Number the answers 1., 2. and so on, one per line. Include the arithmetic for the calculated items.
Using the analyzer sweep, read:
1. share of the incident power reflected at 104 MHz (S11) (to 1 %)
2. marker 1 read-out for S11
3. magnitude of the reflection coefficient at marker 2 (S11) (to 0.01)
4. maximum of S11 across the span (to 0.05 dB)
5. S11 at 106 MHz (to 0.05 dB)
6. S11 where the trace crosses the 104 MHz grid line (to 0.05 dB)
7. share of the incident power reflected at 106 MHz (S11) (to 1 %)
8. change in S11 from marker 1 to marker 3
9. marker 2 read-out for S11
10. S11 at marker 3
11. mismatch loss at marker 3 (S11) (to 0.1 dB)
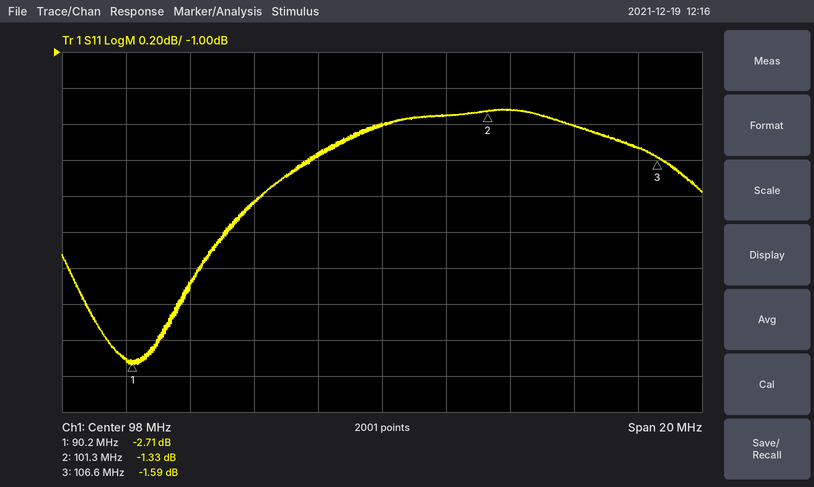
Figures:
1. 10^(-1.4/10) ≈ 72 %
2. -2.71 dB
3. 10^(-1.33/20) ≈ 0.86
4. -1.30 dB
5. -1.55 dB
6. -1.40 dB
7. 10^(-1.55/10) ≈ 70 %
8. -1.59 − (-2.71) = 1.12 dB
9. -1.33 dB
10. -1.59 dB
11. −10 log10(1 − 10^(-1.59/10)) ≈ 5.1 dB
